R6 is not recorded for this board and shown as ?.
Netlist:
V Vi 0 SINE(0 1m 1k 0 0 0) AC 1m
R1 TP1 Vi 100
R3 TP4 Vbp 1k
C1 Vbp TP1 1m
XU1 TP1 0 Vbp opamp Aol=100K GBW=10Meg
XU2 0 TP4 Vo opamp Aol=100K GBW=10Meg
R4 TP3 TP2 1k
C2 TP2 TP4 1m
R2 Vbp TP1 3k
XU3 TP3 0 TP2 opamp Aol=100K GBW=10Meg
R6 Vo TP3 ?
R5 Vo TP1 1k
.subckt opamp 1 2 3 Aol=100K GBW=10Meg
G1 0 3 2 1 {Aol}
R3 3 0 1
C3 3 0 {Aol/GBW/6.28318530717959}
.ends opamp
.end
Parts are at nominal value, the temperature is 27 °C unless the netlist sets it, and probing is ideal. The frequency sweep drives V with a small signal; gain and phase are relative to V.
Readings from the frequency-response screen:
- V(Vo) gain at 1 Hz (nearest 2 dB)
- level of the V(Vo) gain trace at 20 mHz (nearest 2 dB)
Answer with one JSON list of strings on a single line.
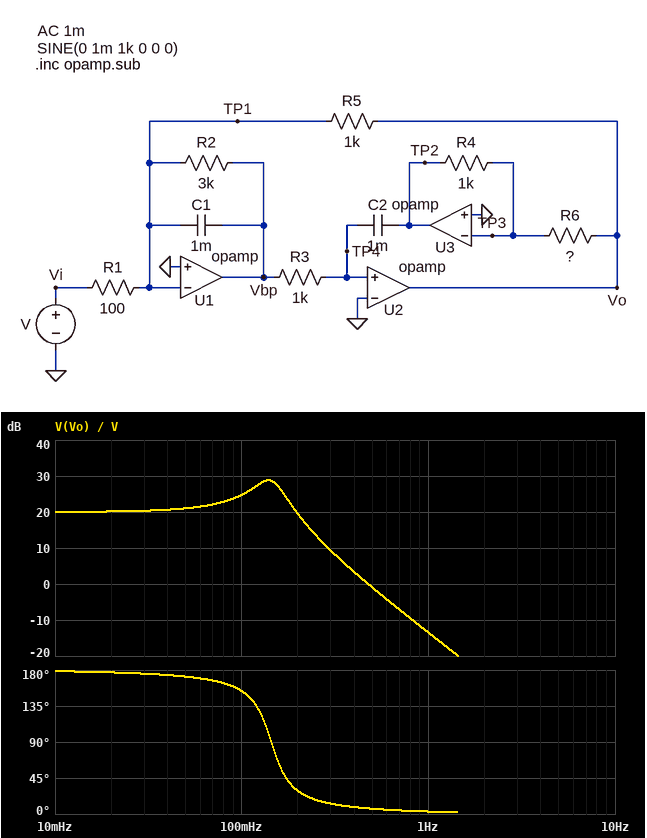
["-14 dB", "20 dB"]
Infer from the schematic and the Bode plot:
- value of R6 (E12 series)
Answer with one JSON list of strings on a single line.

["820 Ω"]
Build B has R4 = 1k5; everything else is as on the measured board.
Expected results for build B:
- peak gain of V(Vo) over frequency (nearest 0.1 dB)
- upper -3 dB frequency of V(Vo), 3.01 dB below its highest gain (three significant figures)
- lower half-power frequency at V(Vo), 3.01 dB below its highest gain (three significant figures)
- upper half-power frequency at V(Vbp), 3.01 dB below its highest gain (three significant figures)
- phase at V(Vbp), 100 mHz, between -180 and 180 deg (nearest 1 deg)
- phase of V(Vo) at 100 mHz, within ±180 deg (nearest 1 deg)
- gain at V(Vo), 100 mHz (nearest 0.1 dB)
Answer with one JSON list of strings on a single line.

["27.1 dB", "136 mHz", "79.7 mHz", "147 mHz", "-144 deg", "126 deg", "26.5 dB"]
